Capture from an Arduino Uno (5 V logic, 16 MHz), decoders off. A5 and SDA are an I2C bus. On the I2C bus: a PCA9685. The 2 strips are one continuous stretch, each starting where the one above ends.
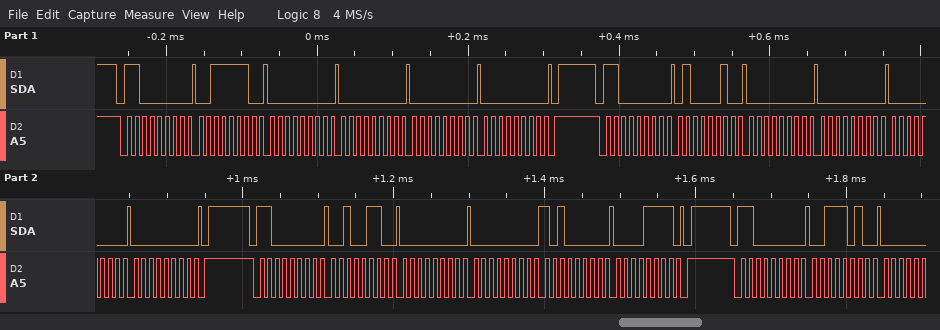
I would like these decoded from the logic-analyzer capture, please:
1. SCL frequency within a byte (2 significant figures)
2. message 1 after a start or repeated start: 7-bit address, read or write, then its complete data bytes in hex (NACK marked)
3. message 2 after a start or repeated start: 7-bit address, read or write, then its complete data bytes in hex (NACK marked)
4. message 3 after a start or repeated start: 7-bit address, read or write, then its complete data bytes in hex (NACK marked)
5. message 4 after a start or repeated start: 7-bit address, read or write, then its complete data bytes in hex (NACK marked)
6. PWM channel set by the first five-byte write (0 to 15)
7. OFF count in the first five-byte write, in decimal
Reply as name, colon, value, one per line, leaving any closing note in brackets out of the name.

SCL frequency within a byte: 100 kHz
message 1 after a start or repeated start: 7-bit address, read or write, then its complete data bytes in hex: 0x60 write: 3E 00 00 00 00
message 2 after a start or repeated start: 7-bit address, read or write, then its complete data bytes in hex: 0x60 write: 42 00 00 00 00
message 3 after a start or repeated start: 7-bit address, read or write, then its complete data bytes in hex: 0x60 write: 26 00 00 A0 0F
message 4 after a start or repeated start: 7-bit address, read or write, then its complete data bytes in hex: 0x60 write: 3A
PWM channel set by the first five-byte write: 14
OFF count in the first five-byte write, in decimal: 0
